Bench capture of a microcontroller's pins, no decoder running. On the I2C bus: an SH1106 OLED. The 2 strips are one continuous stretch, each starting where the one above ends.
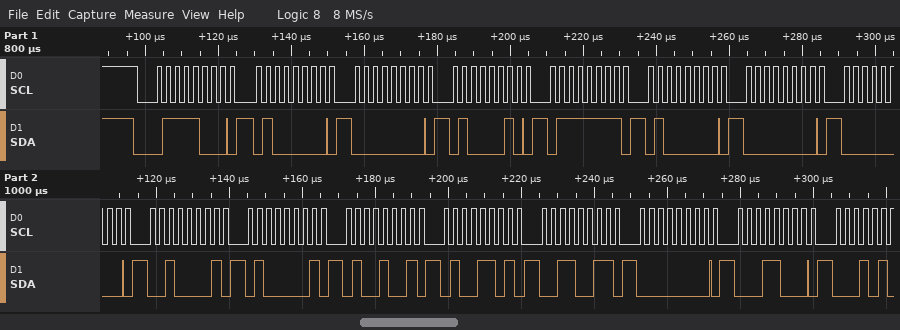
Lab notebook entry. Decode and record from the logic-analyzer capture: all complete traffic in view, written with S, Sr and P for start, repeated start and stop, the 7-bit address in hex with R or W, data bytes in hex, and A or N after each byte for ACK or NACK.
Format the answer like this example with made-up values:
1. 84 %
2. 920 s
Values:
1. S 3CW A 40 A 00 A 42 A 7F A 40 A 00 A 00 A 21 A 41 A 49 A 4D A 33 A 00 A 18 A
